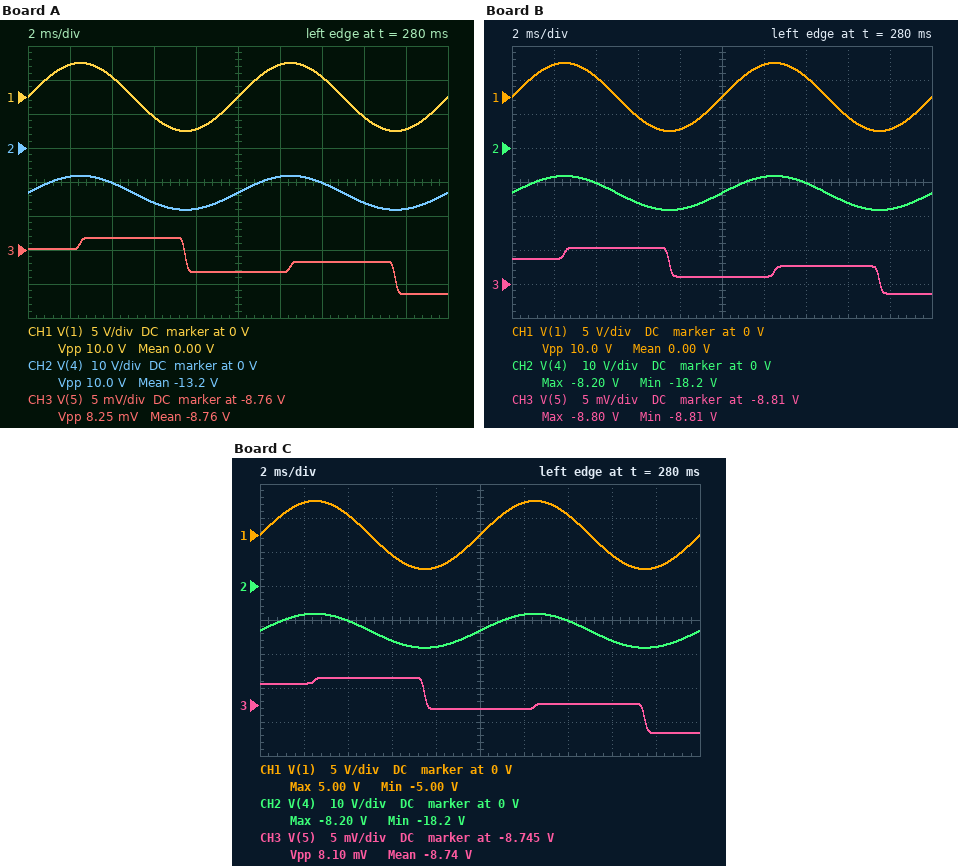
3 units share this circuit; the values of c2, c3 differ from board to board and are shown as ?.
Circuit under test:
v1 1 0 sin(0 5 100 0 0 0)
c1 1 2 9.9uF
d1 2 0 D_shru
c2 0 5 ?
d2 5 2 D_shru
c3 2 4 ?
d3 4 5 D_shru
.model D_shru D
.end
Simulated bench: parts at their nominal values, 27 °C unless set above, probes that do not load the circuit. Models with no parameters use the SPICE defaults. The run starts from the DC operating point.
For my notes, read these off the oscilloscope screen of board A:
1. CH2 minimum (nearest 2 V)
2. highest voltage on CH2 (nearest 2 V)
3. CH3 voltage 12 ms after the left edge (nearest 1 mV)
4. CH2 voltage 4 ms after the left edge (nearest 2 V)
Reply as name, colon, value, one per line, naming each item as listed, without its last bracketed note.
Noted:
CH2 minimum: -18 V
highest voltage on CH2: -8 V
CH3 voltage 12 ms after the left edge: -8.763 V
CH2 voltage 4 ms after the left edge: -10 V
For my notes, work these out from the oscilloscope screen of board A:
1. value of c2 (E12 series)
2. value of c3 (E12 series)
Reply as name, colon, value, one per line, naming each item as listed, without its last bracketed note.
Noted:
value of c2: 15 µF
value of c3: 6.8 µF
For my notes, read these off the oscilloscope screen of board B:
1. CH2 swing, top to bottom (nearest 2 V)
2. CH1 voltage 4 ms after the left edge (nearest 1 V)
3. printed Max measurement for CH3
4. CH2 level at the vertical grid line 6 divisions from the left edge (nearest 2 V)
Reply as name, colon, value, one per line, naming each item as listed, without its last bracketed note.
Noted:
CH2 swing, top to bottom: 10 V
CH1 voltage 4 ms after the left edge: 3 V
printed Max measurement for CH3: -8.80 V
CH2 level at the vertical grid line 6 divisions from the left edge: -8 V
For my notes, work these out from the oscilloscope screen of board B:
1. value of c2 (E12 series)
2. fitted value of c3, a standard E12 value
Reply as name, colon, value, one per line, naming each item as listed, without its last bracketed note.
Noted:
value of c2: 6.8 µF
fitted value of c3, a standard E12 value: 3.9 µF
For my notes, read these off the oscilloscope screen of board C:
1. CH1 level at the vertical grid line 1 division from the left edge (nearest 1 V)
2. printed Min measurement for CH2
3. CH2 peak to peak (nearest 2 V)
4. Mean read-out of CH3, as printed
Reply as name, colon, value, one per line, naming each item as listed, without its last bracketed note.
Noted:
CH1 level at the vertical grid line 1 division from the left edge: 5 V
printed Min measurement for CH2: -18.2 V
CH2 peak to peak: 10 V
Mean read-out of CH3, as printed: -8.74 V
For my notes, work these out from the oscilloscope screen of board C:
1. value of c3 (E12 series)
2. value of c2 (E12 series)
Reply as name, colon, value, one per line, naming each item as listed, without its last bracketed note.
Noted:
value of c3: 4.7 µF
value of c2: 22 µF
